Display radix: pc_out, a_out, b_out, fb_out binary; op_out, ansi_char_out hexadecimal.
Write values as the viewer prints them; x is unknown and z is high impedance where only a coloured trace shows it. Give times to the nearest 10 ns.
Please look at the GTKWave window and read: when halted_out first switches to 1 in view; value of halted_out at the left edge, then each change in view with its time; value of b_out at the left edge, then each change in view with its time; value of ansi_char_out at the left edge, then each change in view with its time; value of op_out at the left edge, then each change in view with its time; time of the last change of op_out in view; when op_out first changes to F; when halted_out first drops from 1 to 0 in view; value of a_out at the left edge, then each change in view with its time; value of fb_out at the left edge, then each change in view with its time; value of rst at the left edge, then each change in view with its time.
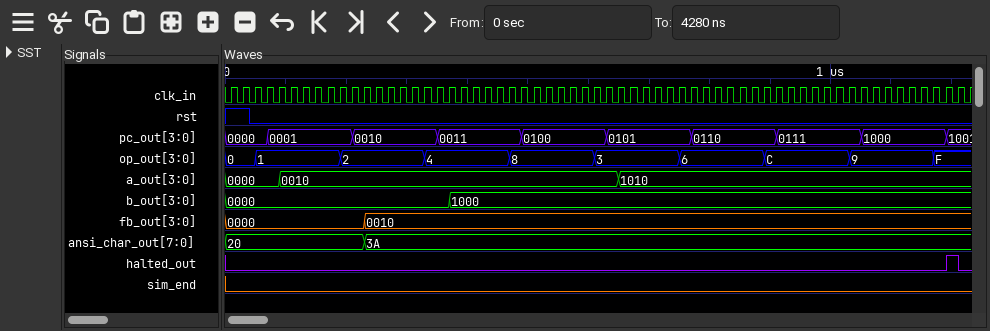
1190 ns
0, 1 at 1190 ns, 0 at 1210 ns
0000, 1000 at 370 ns
20, 3A at 230 ns
0, 1 at 50 ns, 2 at 190 ns, 4 at 330 ns, 8 at 470 ns, 3 at 610 ns, 6 at 750 ns, C at 890 ns, 9 at 1030 ns, F at 1170 ns
1170 ns
1170 ns
1210 ns
0000, 0010 at 90 ns, 1010 at 650 ns
0000, 0010 at 230 ns
1, 0 at 40 ns
